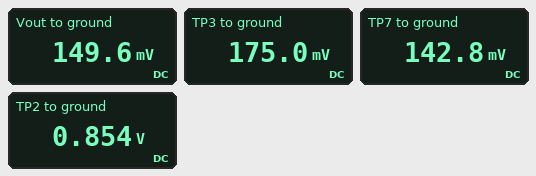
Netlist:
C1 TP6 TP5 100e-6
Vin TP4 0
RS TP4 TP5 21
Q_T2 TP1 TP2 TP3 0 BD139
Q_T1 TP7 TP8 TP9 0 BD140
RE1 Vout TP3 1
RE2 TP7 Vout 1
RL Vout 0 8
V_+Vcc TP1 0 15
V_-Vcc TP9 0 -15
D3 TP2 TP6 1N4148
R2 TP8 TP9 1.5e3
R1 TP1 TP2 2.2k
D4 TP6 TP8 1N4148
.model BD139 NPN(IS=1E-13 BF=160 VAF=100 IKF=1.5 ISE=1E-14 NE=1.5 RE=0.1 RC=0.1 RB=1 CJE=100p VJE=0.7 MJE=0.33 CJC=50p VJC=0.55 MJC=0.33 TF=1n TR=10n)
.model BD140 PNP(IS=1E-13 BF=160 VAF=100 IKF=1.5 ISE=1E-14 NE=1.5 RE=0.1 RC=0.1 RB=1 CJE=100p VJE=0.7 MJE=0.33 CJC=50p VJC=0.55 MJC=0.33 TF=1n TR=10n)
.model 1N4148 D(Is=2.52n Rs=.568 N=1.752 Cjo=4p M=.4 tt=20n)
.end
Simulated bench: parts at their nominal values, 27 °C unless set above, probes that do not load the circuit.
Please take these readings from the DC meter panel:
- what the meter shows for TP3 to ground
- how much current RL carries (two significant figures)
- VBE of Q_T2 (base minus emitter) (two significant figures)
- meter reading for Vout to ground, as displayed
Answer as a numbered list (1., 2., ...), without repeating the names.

1. 175.0 mV
2. 19 mA
3. 680 mV
4. 149.6 mV
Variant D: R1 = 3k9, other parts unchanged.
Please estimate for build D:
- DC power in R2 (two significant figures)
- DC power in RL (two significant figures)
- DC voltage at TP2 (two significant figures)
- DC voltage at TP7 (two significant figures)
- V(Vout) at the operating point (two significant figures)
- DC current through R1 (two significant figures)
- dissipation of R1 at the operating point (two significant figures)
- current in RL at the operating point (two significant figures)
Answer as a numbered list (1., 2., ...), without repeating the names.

1. 140 mW
2. 490 µW
3. 570 mV
4. -74 mV
5. -63 mV
6. 3.7 mA
7. 53 mW
8. 7.8 mA
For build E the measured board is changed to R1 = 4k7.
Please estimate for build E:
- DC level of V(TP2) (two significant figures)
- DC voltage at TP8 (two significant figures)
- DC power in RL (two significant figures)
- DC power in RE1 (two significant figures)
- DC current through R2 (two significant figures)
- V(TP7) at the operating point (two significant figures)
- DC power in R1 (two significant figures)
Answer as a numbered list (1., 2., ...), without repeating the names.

1. 520 mV
2. -750 mV
3. 970 µW
4. 3.3 µW
5. 9.5 mA
6. -100 mV
7. 45 mW
